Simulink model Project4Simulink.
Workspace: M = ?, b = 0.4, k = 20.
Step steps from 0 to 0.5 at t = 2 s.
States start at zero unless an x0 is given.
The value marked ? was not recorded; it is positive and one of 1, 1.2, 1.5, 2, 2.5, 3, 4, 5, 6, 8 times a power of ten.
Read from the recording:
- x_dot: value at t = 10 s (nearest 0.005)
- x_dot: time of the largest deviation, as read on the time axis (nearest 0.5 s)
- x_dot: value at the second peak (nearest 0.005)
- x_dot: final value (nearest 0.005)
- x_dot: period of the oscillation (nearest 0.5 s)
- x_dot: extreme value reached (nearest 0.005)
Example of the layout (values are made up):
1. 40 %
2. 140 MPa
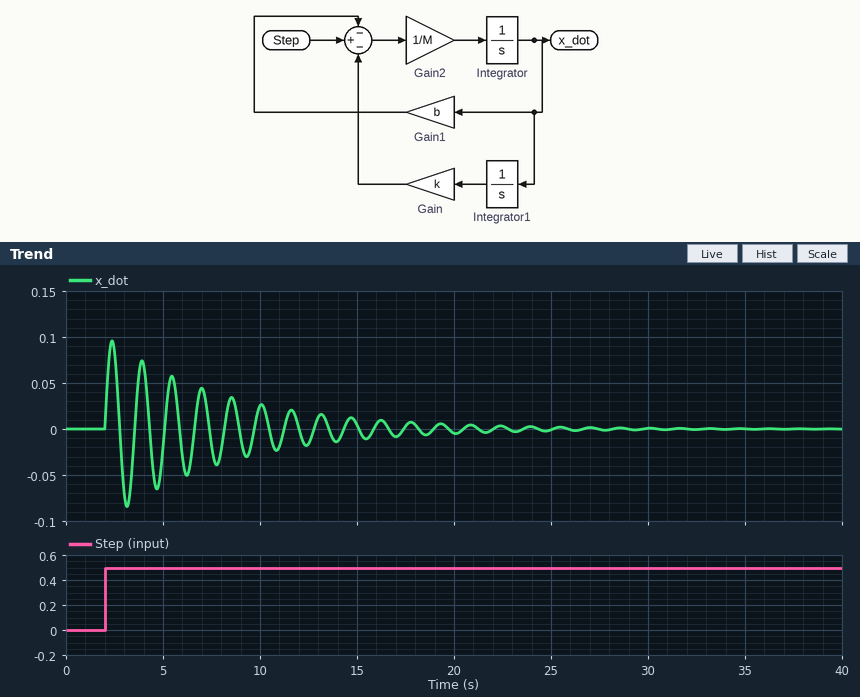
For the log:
1. 0.025
2. 2.5 s
3. 0.075
4. 0.000
5. 1.5 s
6. 0.095
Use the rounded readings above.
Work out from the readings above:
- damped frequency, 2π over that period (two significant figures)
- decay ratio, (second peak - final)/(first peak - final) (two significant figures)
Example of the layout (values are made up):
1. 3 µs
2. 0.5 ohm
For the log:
1. 4.2 rad/s
2. 0.79
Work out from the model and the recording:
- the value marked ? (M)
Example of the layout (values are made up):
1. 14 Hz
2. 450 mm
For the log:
1. 1.2
